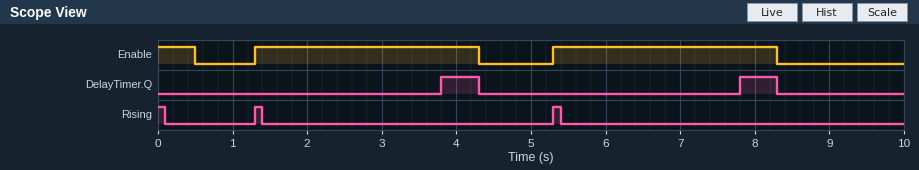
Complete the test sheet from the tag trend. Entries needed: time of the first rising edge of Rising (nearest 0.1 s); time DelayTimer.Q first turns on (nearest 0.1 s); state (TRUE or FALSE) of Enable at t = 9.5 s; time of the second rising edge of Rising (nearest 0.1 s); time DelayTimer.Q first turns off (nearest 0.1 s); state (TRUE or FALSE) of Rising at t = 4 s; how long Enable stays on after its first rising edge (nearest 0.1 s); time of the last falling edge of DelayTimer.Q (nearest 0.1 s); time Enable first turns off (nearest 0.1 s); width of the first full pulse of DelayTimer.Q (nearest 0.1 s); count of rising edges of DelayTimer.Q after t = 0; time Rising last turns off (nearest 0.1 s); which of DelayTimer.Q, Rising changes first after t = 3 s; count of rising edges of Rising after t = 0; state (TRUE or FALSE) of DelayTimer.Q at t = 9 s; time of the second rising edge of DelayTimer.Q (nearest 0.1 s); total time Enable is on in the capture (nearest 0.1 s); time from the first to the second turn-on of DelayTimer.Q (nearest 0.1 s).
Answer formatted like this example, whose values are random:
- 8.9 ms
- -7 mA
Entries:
- 1.3 s
- 3.8 s
- FALSE
- 5.3 s
- 4.3 s
- FALSE
- 3.0 s
- 8.3 s
- 0.5 s
- 0.5 s
- 2
- 5.4 s
- DelayTimer.Q
- 2
- FALSE
- 7.8 s
- 6.5 s
- 4.0 s
